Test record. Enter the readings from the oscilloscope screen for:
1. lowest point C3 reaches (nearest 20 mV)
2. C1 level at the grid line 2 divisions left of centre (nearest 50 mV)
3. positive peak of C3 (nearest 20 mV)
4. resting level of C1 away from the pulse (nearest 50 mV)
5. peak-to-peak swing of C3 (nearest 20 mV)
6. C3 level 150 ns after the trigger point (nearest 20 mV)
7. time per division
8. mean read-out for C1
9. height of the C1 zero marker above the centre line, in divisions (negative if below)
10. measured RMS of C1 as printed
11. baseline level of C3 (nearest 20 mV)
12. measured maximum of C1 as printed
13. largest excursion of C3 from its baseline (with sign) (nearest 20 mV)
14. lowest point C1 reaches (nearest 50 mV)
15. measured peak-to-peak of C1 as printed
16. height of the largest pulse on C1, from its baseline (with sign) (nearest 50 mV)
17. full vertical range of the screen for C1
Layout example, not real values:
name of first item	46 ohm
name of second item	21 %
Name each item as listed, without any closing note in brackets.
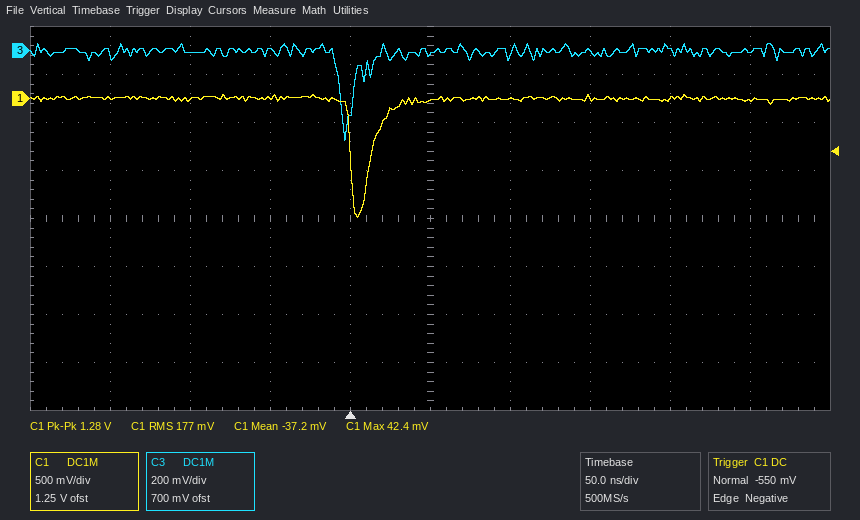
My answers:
lowest point C3 reaches	-380 mV
C1 level at the grid line 2 divisions left of centre	0 mV
positive peak of C3	20 mV
resting level of C1 away from the pulse	0 mV
peak-to-peak swing of C3	400 mV
C3 level 150 ns after the trigger point	0 mV
time per division	50 ns
mean read-out for C1	-37.2 mV
height of the C1 zero marker above the centre line, in divisions	+2.5 div
measured RMS of C1 as printed	177 mV
baseline level of C3	0 mV
measured maximum of C1 as printed	42.4 mV
largest excursion of C3 from its baseline (with sign)	-380 mV
lowest point C1 reaches	-1.25 V
measured peak-to-peak of C1 as printed	1.28 V
height of the largest pulse on C1, from its baseline (with sign)	-1.25 V
full vertical range of the screen for C1	4 V
